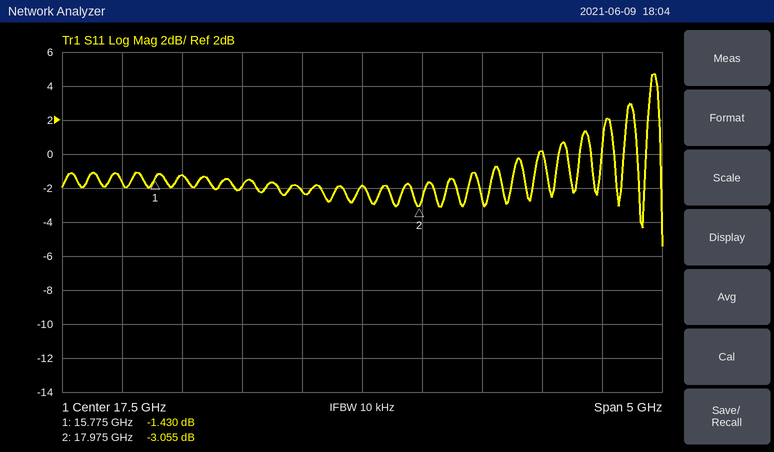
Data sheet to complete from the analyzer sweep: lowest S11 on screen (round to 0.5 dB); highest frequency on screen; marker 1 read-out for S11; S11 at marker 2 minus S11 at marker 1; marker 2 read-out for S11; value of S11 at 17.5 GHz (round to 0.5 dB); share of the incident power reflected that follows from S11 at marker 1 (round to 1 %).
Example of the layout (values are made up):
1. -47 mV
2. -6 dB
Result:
1. -5.5 dB
2. 20 GHz
3. -1.430 dB
4. -1.625 dB
5. -3.055 dB
6. -2.0 dB
7. 72 %
